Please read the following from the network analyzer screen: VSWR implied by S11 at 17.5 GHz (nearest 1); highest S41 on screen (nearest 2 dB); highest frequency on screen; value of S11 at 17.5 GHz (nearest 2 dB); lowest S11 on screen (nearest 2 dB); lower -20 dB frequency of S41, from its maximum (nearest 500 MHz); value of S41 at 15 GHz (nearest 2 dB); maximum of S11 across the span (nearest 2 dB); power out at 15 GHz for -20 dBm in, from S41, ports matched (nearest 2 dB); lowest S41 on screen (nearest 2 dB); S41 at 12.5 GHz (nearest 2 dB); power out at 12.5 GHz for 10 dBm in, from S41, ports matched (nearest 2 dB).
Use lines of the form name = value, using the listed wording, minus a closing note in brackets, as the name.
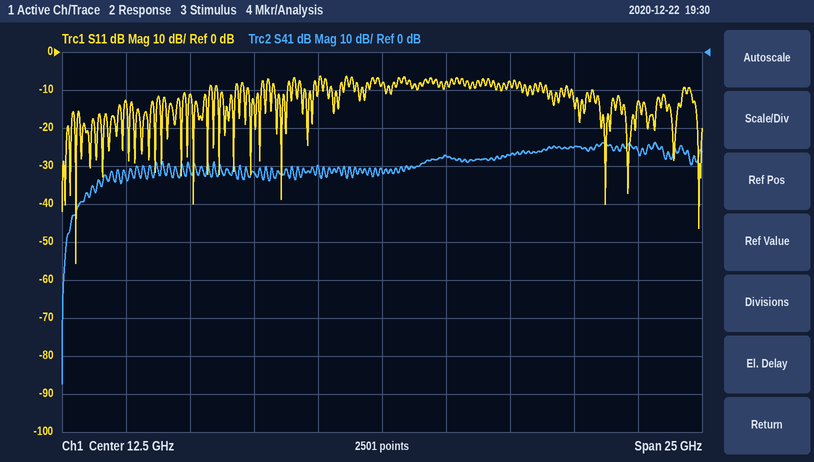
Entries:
VSWR implied by S11 at 17.5 GHz = 2
highest S41 on screen = -24 dB
highest frequency on screen = 25 GHz
value of S11 at 17.5 GHz = -8 dB
lowest S11 on screen = -56 dB
lower -20 dB frequency of S41, from its maximum = 500 MHz
value of S41 at 15 GHz = -28 dB
maximum of S11 across the span = -6 dB
power out at 15 GHz for -20 dBm in, from S41, ports matched = -48 dBm
lowest S41 on screen = -88 dB
S41 at 12.5 GHz = -32 dB
power out at 12.5 GHz for 10 dBm in, from S41, ports matched = -22 dBm
